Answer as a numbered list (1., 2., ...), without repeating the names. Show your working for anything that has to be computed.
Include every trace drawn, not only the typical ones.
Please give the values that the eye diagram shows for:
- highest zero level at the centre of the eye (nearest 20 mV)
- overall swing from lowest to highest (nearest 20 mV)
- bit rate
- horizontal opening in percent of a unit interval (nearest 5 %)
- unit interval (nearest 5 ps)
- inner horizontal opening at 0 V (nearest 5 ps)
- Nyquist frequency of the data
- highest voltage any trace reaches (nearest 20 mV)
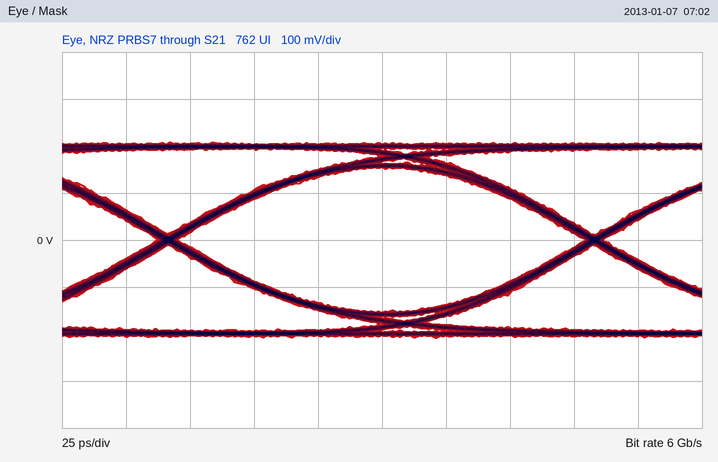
1. -160 mV
2. 420 mV
3. 6 Gb/s
4. 160 ps / 165 ps ≈ 97.0 %, so 95 % to the nearest 5 %
5. 165 ps
6. 160 ps
7. 3 GHz
8. 200 mV
